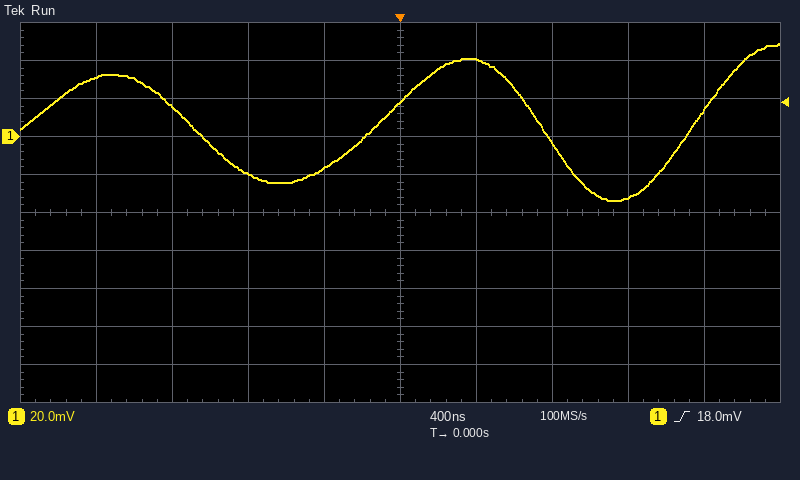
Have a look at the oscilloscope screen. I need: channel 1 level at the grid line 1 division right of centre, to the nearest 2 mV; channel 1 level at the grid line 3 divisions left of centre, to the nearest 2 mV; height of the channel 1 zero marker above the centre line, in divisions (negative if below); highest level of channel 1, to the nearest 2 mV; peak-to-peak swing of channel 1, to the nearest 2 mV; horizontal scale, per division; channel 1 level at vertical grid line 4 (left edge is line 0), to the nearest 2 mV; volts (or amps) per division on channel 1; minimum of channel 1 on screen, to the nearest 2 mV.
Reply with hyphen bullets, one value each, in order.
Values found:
- 40 mV
- 16 mV
- +2.0 div
- 48 mV
- 82 mV
- 400 ns
- -16 mV
- 20 mV
- -34 mV
